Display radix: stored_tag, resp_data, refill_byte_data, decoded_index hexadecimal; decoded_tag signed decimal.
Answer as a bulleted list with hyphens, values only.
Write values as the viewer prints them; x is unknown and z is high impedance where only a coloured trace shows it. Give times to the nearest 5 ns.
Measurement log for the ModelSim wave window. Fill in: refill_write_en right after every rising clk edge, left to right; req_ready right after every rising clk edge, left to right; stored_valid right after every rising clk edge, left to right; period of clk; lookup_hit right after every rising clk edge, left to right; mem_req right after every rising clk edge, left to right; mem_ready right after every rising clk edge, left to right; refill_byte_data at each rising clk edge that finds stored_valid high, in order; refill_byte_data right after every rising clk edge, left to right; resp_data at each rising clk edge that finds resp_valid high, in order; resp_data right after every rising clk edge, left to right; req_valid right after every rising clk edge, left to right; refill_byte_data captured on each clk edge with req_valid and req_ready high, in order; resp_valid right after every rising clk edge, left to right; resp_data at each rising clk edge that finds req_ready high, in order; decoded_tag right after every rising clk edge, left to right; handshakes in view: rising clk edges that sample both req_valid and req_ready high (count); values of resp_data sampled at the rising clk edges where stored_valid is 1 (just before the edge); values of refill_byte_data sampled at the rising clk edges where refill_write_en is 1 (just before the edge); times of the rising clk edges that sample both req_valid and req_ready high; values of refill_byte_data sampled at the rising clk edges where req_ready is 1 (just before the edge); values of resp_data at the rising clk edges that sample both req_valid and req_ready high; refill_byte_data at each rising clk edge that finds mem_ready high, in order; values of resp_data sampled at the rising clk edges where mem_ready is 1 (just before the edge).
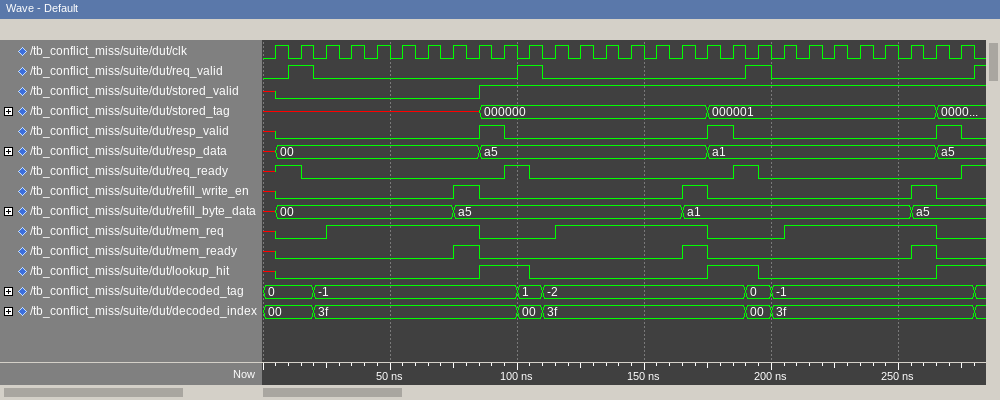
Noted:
- 0 0 0 0 0 0 0 1 0 0 0 0 0 0 0 0 1 0 0 0 0 0 0 0 0 1 0 0
- 1 0 0 0 0 0 0 0 0 1 0 0 0 0 0 0 0 0 1 0 0 0 0 0 0 0 0 1
- 0 0 0 0 0 0 0 0 1 1 1 1 1 1 1 1 1 1 1 1 1 1 1 1 1 1 1 1
- 10 ns
- 0 0 0 0 0 0 0 0 1 1 0 0 0 0 0 0 0 1 1 0 0 0 0 0 0 0 1 1
- 0 0 1 1 1 1 1 1 0 0 0 1 1 1 1 1 1 0 0 0 1 1 1 1 1 1 0 0
- 0 0 0 0 0 0 0 1 0 0 0 0 0 0 0 0 1 0 0 0 0 0 0 0 0 1 0 0
- a5, a5, a5, a5, a5, a5, a5, a5, a1, a1, a1, a1, a1, a1, a1, a1, a1, a5, a5
- 00, 00, 00, 00, 00, 00, 00, a5, a5, a5, a5, a5, a5, a5, a5, a5, a1, a1, a1, a1, a1, a1, a1, a1, a1, a5, a5, a5
- a5, a1, a5
- 00, 00, 00, 00, 00, 00, 00, 00, a5, a5, a5, a5, a5, a5, a5, a5, a5, a1, a1, a1, a1, a1, a1, a1, a1, a1, a5, a5
- 0 1 0 0 0 0 0 0 0 0 1 0 0 0 0 0 0 0 0 1 0 0 0 0 0 0 0 0
- 00, a5, a1
- 0 0 0 0 0 0 0 0 1 0 0 0 0 0 0 0 0 1 0 0 0 0 0 0 0 0 1 0
- 00, a5, a1
- 0, 0, -1, -1, -1, -1, -1, -1, -1, -1, 1, -2, -2, -2, -2, -2, -2, -2, -2, 0, -1, -1, -1, -1, -1, -1, -1, -1
- 3
- a5, a5, a5, a5, a5, a5, a5, a5, a5, a1, a1, a1, a1, a1, a1, a1, a1, a1, a5
- a5, a1, a5
- 15 ns, 105 ns, 195 ns
- 00, a5, a1
- 00, a5, a1
- a5, a1, a5
- 00, a5, a1
